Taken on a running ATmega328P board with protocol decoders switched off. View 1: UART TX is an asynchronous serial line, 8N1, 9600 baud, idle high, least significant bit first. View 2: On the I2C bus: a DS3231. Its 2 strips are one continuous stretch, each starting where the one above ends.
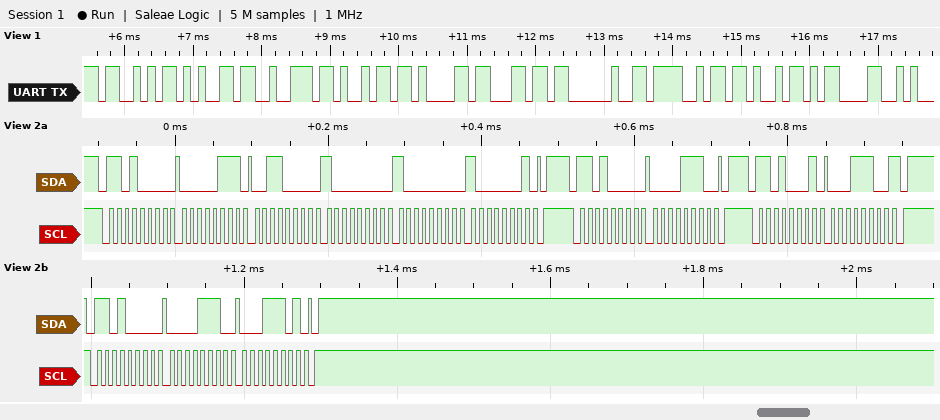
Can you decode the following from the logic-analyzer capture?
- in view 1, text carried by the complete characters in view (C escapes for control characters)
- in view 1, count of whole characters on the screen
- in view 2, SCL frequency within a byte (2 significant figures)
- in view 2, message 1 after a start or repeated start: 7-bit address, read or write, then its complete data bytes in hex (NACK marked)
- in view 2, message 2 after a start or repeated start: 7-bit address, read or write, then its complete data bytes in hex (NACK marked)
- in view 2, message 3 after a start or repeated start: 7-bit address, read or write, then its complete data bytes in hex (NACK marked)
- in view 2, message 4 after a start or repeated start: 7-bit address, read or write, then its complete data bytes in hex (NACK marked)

"Serial OK\r"
10
100 kHz
0x68 write: 07 30 80 80 81
0x68 write: 0E
0x68 read: 1C NACK
0x68 write: 0E 1D
